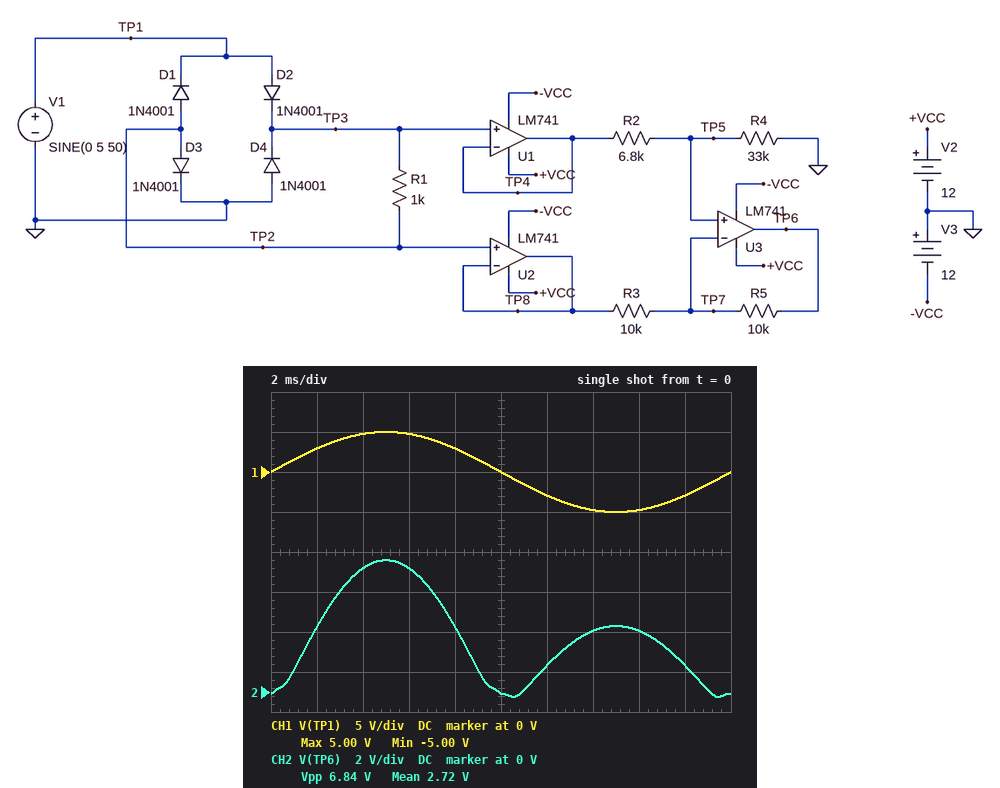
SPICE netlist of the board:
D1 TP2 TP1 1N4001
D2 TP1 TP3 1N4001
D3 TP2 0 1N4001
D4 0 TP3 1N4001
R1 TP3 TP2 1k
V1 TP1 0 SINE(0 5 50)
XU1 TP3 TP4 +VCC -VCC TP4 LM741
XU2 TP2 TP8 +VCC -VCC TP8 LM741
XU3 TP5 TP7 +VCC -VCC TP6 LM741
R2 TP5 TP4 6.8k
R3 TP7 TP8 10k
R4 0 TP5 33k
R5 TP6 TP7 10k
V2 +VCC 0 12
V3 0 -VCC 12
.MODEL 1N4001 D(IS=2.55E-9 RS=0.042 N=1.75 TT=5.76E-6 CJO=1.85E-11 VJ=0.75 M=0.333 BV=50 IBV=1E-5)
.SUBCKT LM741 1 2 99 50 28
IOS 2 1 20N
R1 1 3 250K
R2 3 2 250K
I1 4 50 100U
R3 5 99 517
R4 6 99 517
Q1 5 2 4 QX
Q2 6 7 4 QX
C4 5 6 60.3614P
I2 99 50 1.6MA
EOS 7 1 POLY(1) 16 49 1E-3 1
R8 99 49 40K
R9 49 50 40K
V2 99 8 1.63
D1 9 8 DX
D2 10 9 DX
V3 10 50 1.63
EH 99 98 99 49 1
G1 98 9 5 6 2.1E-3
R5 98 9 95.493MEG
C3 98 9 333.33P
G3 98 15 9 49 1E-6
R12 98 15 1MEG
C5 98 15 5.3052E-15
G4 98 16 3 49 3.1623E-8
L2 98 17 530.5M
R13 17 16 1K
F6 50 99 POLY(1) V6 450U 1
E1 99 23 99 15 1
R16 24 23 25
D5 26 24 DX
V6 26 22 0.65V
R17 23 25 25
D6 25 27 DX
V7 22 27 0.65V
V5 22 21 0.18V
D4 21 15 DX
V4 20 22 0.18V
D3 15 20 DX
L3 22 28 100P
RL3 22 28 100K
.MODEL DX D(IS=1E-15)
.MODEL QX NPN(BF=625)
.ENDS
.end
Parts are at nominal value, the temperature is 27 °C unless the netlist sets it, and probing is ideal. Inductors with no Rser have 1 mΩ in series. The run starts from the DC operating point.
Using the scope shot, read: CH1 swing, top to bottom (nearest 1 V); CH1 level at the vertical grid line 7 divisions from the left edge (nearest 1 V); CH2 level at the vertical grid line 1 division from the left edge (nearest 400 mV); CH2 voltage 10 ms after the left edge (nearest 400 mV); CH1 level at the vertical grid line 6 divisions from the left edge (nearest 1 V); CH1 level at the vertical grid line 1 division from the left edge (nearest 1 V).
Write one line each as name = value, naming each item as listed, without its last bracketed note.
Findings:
CH1 swing, top to bottom = 10 V
CH1 level at the vertical grid line 7 divisions from the left edge = -5 V
CH2 level at the vertical grid line 1 division from the left edge = 3.2 V
CH2 voltage 10 ms after the left edge = 0 V
CH1 level at the vertical grid line 6 divisions from the left edge = -3 V
CH1 level at the vertical grid line 1 division from the left edge = 3 V
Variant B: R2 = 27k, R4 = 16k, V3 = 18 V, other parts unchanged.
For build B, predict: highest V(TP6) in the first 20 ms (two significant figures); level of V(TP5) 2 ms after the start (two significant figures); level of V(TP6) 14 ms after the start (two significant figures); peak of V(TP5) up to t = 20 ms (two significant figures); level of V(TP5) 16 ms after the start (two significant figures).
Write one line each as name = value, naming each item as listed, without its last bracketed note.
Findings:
highest V(TP6) in the first 20 ms = 3.9 V
level of V(TP5) 2 ms after the start = 870 mV
level of V(TP6) 14 ms after the start = 3.6 V
peak of V(TP5) up to t = 20 ms = 1.6 V
level of V(TP5) 16 ms after the start = -240 mV
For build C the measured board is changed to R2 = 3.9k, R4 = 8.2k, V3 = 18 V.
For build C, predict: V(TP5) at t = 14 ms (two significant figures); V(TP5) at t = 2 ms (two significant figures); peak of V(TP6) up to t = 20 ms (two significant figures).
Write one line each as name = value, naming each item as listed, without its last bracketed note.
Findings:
V(TP5) at t = 14 ms = -430 mV
V(TP5) at t = 2 ms = 1.6 V
peak of V(TP6) up to t = 20 ms = 5.3 V
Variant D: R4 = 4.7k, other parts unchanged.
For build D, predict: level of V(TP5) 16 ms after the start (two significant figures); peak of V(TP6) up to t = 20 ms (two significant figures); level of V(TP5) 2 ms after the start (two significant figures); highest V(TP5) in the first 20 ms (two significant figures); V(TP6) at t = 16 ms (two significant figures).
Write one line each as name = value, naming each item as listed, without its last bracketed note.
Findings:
level of V(TP5) 16 ms after the start = -260 mV
peak of V(TP6) up to t = 20 ms = 3.8 V
level of V(TP5) 2 ms after the start = 950 mV
highest V(TP5) in the first 20 ms = 1.8 V
V(TP6) at t = 16 ms = 3.6 V
